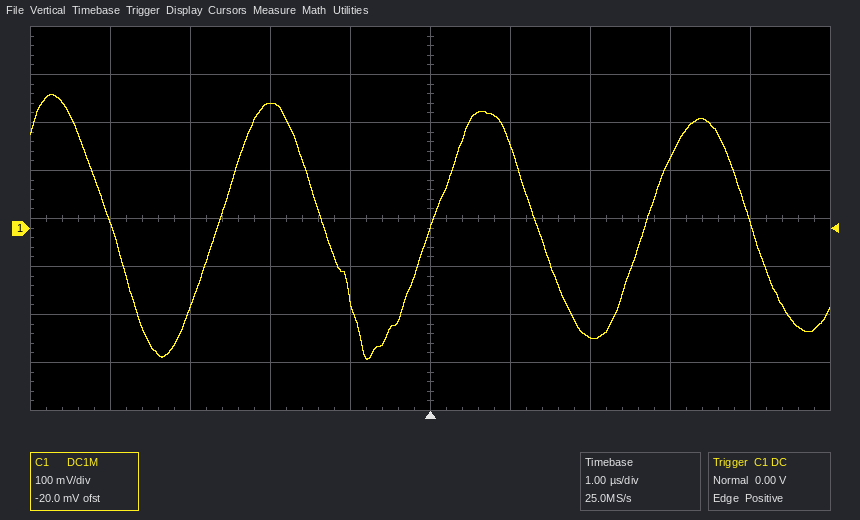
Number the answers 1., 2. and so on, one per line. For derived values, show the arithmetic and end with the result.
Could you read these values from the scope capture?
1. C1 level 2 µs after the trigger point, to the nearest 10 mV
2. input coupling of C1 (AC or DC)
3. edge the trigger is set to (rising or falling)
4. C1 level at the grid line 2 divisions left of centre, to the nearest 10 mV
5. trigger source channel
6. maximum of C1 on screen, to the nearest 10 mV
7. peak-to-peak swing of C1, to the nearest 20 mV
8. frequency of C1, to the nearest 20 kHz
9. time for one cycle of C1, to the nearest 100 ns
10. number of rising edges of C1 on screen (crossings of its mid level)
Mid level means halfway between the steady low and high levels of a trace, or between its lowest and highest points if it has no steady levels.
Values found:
1. -230 mV
2. DC
3. rising
4. 260 mV
5. C1
6. 280 mV
7. 560 mV
8. 1 / 2.7 µs ≈ 370 kHz, so 380 kHz to the nearest 20 kHz
9. 2.7 µs
10. 3
